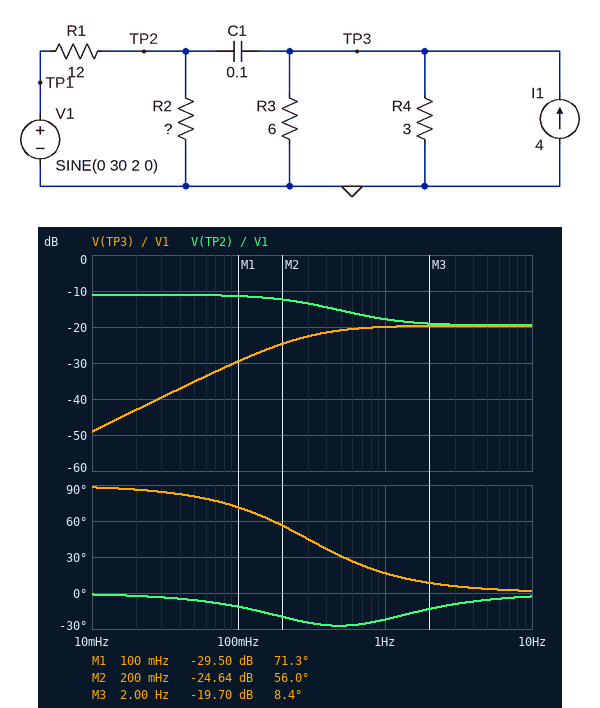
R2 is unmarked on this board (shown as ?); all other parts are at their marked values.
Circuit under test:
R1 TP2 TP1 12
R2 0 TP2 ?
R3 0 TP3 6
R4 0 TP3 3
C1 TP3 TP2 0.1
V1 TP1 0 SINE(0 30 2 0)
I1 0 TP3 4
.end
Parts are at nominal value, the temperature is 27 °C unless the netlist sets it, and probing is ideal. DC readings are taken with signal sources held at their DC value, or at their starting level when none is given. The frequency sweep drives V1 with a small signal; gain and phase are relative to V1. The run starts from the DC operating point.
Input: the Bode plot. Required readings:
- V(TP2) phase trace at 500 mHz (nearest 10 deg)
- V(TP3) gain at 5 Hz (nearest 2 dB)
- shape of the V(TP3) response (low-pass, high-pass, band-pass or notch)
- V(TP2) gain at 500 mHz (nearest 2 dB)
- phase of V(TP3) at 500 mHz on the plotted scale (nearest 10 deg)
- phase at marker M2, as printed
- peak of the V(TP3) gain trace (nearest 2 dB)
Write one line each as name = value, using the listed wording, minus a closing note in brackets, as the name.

V(TP2) phase trace at 500 mHz = -30 deg
V(TP3) gain at 5 Hz = -20 dB
shape of the V(TP3) response = high-pass
V(TP2) gain at 500 mHz = -16 dB
phase of V(TP3) at 500 mHz on the plotted scale = 30 deg
phase at marker M2, as printed = 56.0 deg
peak of the V(TP3) gain trace = -20 dB
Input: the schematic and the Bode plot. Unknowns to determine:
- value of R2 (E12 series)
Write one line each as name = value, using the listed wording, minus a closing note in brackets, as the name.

value of R2 = 4.7 Ω
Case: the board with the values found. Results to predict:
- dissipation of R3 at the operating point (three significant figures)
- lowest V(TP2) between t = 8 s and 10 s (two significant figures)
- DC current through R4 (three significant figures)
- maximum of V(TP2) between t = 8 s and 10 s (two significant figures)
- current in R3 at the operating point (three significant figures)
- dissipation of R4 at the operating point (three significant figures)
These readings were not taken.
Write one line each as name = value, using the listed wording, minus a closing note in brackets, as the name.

dissipation of R3 at the operating point = 10.7 W
lowest V(TP2) between t = 8 s and 10 s = -3.3 V
DC current through R4 = 2.67 A
maximum of V(TP2) between t = 8 s and 10 s = 3.3 V
current in R3 at the operating point = 1.33 A
dissipation of R4 at the operating point = 21.3 W
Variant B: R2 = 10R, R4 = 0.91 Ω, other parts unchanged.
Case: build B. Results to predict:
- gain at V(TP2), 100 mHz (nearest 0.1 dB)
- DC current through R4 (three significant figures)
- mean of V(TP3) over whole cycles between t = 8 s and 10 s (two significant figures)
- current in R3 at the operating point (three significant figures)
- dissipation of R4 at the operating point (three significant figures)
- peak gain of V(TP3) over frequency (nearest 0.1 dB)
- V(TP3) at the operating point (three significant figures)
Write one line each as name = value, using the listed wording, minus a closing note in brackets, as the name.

gain at V(TP2), 100 mHz = -7.5 dB
DC current through R4 = 3.47 A
mean of V(TP3) over whole cycles between t = 8 s and 10 s = 3.2 V
current in R3 at the operating point = 527 mA
dissipation of R4 at the operating point = 11.0 W
peak gain of V(TP3) over frequency = -24.8 dB
V(TP3) at the operating point = 3.16 V
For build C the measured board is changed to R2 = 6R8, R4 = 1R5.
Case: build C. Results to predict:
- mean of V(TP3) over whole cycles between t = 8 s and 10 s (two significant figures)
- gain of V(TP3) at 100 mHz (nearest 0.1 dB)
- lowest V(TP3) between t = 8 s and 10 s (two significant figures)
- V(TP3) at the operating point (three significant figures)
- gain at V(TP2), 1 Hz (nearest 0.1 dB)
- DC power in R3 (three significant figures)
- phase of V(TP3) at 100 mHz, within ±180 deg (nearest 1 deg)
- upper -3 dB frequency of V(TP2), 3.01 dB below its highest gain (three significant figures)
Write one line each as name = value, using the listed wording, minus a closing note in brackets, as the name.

mean of V(TP3) over whole cycles between t = 8 s and 10 s = 4.8 V
gain of V(TP3) at 100 mHz = -31.8 dB
lowest V(TP3) between t = 8 s and 10 s = 2.5 V
V(TP3) at the operating point = 4.80 V
gain at V(TP2), 1 Hz = -18.1 dB
DC power in R3 = 3.84 W
phase of V(TP3) at 100 mHz, within ±180 deg = 71 deg
upper -3 dB frequency of V(TP2), 3.01 dB below its highest gain = 302 mHz
